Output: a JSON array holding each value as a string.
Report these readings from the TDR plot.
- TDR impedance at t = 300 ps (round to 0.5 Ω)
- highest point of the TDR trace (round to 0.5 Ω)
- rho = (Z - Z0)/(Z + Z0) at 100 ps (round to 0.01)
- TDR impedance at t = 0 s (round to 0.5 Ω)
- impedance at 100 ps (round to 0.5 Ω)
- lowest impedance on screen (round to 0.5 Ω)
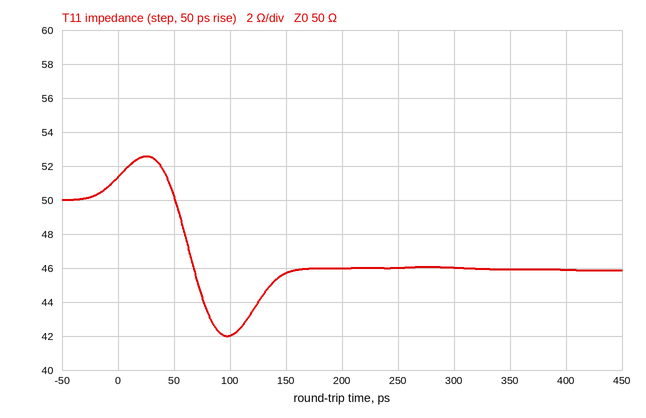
["46.0 Ω", "52.5 Ω", "-0.09", "51.5 Ω", "42.0 Ω", "42.0 Ω"]
